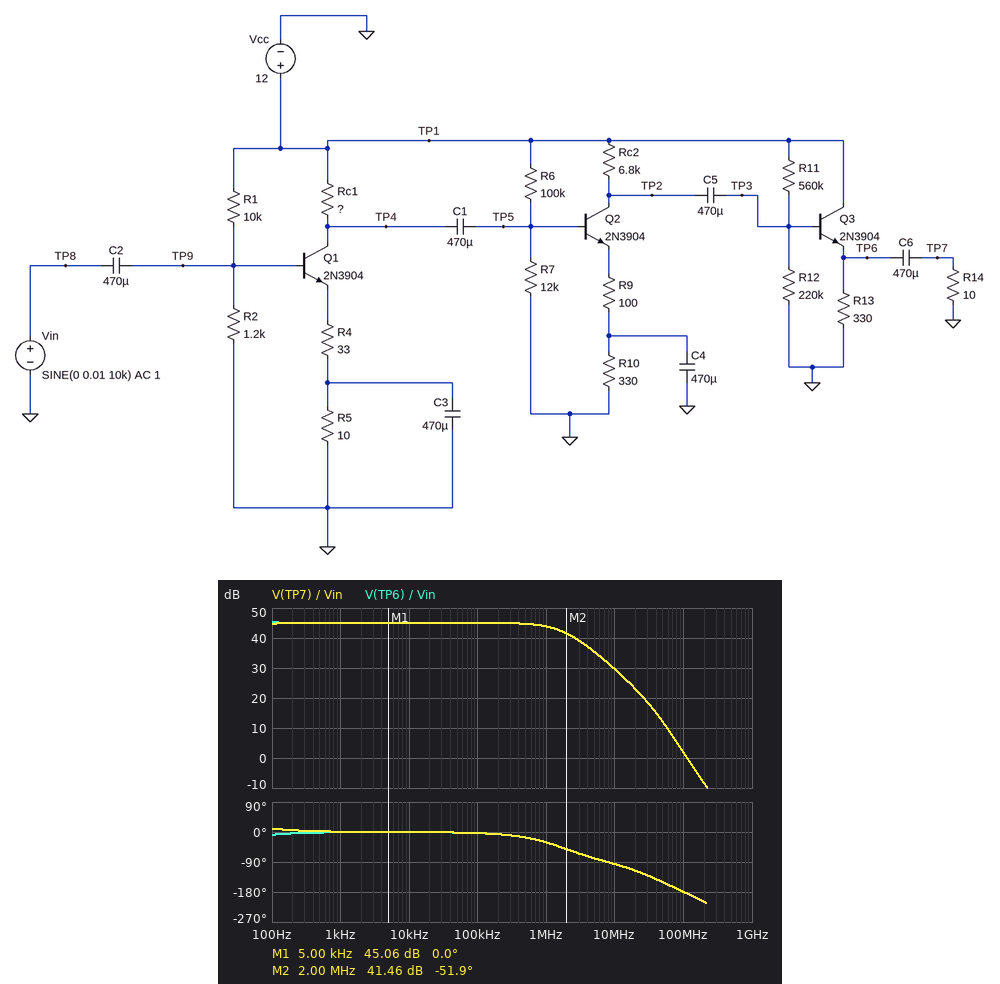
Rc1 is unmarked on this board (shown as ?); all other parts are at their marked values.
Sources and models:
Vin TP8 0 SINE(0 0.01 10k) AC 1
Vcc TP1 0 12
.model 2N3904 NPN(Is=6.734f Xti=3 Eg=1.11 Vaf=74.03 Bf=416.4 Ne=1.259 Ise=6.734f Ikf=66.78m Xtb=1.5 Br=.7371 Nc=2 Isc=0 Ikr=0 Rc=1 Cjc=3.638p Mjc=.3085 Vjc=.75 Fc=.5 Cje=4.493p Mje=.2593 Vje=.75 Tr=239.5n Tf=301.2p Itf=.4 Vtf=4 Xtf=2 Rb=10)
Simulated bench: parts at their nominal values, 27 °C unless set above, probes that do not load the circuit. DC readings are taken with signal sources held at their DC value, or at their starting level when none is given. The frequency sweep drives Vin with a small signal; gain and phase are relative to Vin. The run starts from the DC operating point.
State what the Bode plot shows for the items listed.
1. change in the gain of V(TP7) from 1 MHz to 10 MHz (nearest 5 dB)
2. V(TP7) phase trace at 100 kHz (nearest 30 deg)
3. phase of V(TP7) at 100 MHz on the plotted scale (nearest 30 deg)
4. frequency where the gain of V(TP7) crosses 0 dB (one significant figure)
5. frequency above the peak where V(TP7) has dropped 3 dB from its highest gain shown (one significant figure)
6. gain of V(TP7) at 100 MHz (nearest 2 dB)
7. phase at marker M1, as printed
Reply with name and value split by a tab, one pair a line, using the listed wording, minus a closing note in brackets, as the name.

change in the gain of V(TP7) from 1 MHz to 10 MHz	-15 dB
V(TP7) phase trace at 100 kHz	0 deg
phase of V(TP7) at 100 MHz on the plotted scale	-180 deg
frequency where the gain of V(TP7) crosses 0 dB	100 MHz
frequency above the peak where V(TP7) has dropped 3 dB from its highest gain shown	2 MHz
gain of V(TP7) at 100 MHz	2 dB
phase at marker M1, as printed	0.0 deg
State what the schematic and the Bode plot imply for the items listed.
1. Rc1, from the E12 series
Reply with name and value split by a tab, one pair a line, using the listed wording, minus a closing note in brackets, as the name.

Rc1, from the E12 series	820 Ω
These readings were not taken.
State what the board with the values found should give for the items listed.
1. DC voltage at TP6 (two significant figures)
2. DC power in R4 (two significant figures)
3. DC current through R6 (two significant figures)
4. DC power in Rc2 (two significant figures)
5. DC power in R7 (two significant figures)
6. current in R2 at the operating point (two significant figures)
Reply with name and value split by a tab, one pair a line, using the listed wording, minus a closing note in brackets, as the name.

DC voltage at TP6	690 mV
DC power in R4	4.1 mW
DC current through R6	110 µA
DC power in Rc2	9.9 mW
DC power in R7	120 µW
current in R2 at the operating point	1.0 mA
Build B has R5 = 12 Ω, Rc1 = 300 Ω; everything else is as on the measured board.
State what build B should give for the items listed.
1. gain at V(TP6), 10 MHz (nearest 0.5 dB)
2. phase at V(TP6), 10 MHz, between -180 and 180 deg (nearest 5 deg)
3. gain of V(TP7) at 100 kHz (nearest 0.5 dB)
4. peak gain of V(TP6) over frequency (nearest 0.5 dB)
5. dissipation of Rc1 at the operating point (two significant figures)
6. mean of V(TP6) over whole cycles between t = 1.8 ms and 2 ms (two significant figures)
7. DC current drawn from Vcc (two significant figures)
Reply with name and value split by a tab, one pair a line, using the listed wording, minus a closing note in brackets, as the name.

gain at V(TP6), 10 MHz	24.0 dB
phase at V(TP6), 10 MHz, between -180 and 180 deg	-85 deg
gain of V(TP7) at 100 kHz	37.0 dB
peak gain of V(TP6) over frequency	45.0 dB
dissipation of Rc1 at the operating point	35 mW
mean of V(TP6) over whole cycles between t = 1.8 ms and 2 ms	980 mV
DC current drawn from Vcc	15 mA
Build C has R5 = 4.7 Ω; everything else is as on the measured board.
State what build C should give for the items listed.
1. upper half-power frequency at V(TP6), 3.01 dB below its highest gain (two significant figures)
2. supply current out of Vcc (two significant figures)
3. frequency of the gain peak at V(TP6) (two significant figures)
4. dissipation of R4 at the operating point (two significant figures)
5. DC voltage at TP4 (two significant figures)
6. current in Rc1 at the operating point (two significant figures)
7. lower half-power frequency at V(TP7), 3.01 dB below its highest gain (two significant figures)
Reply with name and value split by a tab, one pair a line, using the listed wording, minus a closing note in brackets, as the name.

upper half-power frequency at V(TP6), 3.01 dB below its highest gain	13 Hz
supply current out of Vcc	17 mA
frequency of the gain peak at V(TP6)	4.8 Hz
dissipation of R4 at the operating point	5.1 mW
DC voltage at TP4	1.9 V
current in Rc1 at the operating point	12 mA
lower half-power frequency at V(TP7), 3.01 dB below its highest gain	10 Hz
